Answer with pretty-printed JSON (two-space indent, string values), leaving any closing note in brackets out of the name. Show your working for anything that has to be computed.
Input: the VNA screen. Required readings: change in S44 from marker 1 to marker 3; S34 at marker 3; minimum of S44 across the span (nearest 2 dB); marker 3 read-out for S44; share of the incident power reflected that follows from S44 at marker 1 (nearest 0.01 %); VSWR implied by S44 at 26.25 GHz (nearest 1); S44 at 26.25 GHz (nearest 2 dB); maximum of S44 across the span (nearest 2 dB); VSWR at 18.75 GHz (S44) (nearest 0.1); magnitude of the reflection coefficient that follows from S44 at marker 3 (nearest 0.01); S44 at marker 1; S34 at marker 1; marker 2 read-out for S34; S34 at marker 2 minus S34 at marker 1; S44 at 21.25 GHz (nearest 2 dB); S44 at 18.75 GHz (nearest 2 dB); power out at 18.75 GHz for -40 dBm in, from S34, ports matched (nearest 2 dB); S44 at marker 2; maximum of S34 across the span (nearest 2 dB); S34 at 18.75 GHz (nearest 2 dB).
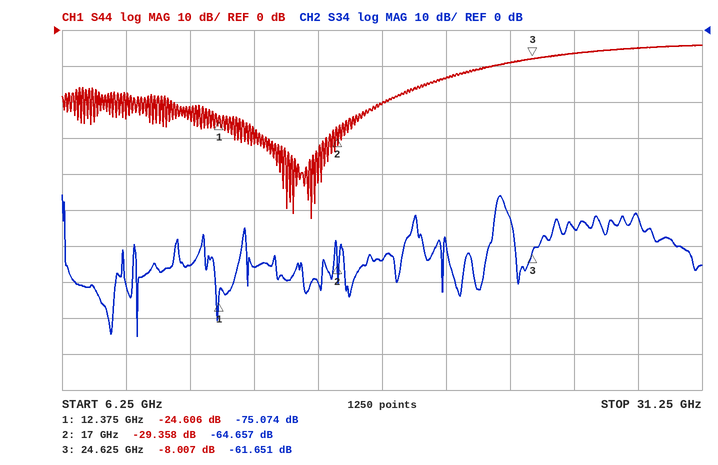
{
  "change in S44 from marker 1 to marker 3": "-8.007 − (-24.606) = 16.599 dB",
  "S34 at marker 3": "-61.651 dB",
  "minimum of S44 across the span": "-52 dB",
  "marker 3 read-out for S44": "-8.007 dB",
  "share of the incident power reflected that follows from S44 at marker 1": "10^(-24.606/10) ≈ 0.35 %",
  "VSWR implied by S44 at 26.25 GHz": "|Γ| = 10^(-6/20) = 0.5012; VSWR = (1 + 0.5012)/(1 − 0.5012) ≈ 3",
  "S44 at 26.25 GHz": "-6 dB",
  "maximum of S44 across the span": "-4 dB",
  "VSWR at 18.75 GHz (S44)": "|Γ| = 10^(-20/20) = 0.1000; VSWR = (1 + 0.1000)/(1 − 0.1000) ≈ 1.2",
  "magnitude of the reflection coefficient that follows from S44 at marker 3": "10^(-8.007/20) ≈ 0.40",
  "S44 at marker 1": "-24.606 dB",
  "S34 at marker 1": "-75.074 dB",
  "marker 2 read-out for S34": "-64.657 dB",
  "S34 at marker 2 minus S34 at marker 1": "-64.657 − (-75.074) = 10.417 dB",
  "S44 at 21.25 GHz": "-14 dB",
  "S44 at 18.75 GHz": "-20 dB",
  "power out at 18.75 GHz for -40 dBm in, from S34, ports matched": "-40 dBm + (-64 dB) = -104 dBm",
  "S44 at marker 2": "-29.358 dB",
  "maximum of S34 across the span": "-46 dB",
  "S34 at 18.75 GHz": "-64 dB"
}
